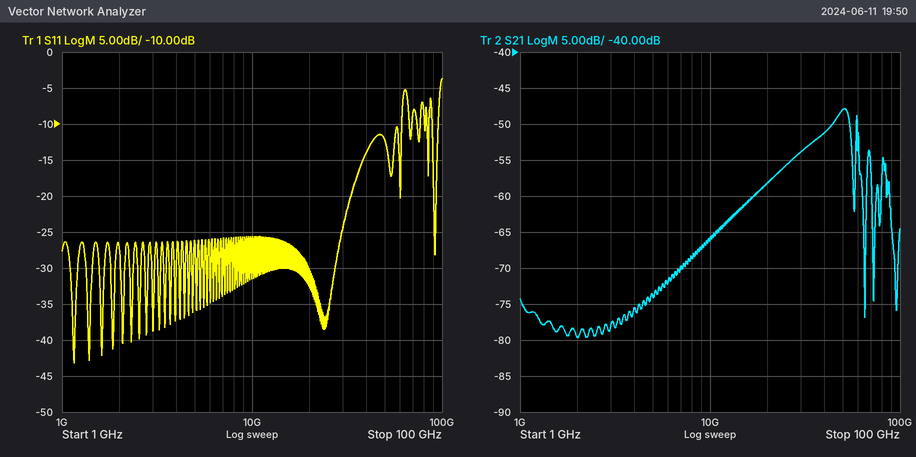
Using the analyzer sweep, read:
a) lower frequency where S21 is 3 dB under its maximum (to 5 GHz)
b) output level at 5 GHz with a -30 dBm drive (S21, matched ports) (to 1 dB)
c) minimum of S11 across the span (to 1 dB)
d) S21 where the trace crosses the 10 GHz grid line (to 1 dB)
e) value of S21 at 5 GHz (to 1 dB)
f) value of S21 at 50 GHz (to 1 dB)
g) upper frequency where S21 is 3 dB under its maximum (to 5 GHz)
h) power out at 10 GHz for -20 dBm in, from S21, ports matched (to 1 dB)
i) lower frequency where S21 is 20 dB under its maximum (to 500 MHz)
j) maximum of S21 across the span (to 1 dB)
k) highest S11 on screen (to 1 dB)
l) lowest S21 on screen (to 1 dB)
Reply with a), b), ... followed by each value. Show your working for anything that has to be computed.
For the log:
a) 40 GHz
b) -30 dBm + (-74 dB) = -104 dBm
c) -43 dB
d) -66 dB
e) -74 dB
f) -48 dB
g) 55 GHz
h) -20 dBm + (-66 dB) = -86 dBm
i) 8.5 GHz
j) -48 dB
k) -4 dB
l) -80 dB
